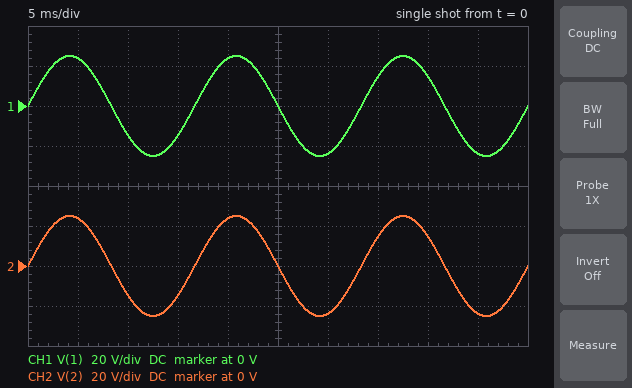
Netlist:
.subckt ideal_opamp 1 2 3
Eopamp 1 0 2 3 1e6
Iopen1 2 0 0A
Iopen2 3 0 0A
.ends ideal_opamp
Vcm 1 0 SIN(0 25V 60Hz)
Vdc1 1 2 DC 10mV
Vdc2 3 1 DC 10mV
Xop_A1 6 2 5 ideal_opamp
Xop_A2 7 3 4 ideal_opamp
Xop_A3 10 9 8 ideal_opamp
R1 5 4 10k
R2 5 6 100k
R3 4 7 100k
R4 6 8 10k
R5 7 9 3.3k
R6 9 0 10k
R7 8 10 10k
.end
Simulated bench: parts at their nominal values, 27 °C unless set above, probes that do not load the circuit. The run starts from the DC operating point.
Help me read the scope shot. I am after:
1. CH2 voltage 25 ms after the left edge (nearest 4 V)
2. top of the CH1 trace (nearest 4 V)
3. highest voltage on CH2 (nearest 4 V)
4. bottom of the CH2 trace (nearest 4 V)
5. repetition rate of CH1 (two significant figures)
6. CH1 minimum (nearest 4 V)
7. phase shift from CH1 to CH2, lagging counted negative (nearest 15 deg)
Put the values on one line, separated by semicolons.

0 V; 24 V; 24 V; -24 V; 60 Hz; -24 V; 0 deg
